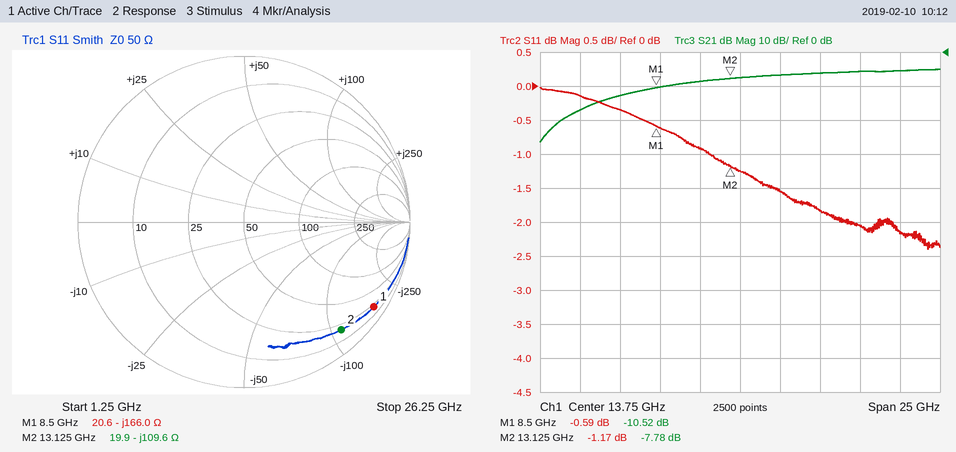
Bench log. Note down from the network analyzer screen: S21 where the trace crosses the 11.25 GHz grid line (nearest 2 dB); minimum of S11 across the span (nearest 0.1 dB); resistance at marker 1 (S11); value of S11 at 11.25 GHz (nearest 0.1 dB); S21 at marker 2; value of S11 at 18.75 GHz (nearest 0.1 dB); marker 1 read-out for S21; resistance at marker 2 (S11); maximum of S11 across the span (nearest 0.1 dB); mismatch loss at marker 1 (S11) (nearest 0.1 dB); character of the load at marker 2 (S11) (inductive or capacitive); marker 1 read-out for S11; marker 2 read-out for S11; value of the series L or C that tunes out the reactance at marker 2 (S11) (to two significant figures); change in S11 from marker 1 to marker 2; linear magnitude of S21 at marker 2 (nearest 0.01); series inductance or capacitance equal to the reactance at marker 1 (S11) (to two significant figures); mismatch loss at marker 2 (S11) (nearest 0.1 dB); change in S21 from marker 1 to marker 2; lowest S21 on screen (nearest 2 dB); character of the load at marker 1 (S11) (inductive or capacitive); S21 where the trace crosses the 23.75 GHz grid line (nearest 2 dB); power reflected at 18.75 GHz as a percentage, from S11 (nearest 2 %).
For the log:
-8 dB
-2.4 dB
20.6 Ω
-0.9 dB
-7.78 dB
-1.8 dB
-10.52 dB
19.9 Ω
0.0 dB
9.0 dB
capacitive
-0.59 dB
-1.17 dB
1.3 nH
-0.58 dB
0.41
110 fF
6.3 dB
2.74 dB
-26 dB
capacitive
-6 dB
66 %
